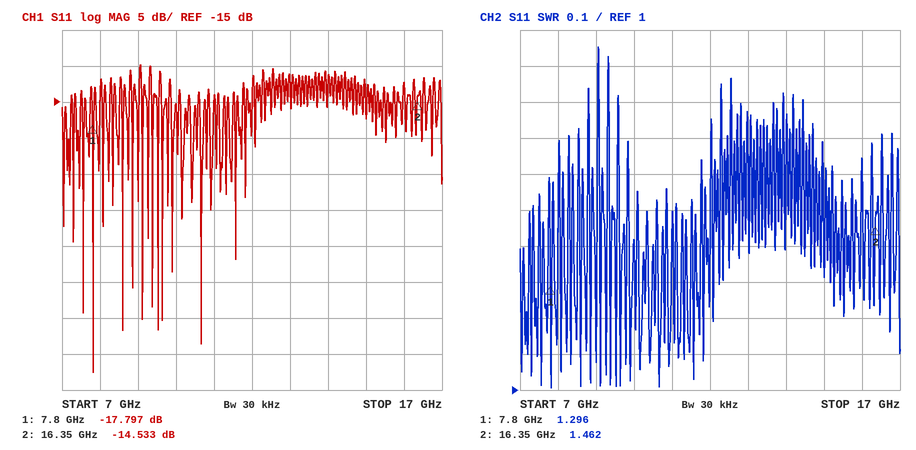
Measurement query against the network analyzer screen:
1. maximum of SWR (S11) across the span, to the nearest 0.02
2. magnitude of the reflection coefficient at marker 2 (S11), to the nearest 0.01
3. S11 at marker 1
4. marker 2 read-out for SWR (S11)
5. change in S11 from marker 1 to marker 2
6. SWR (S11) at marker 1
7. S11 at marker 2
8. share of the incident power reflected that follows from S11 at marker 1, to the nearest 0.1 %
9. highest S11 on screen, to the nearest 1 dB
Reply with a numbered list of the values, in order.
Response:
1. 1.96
2. 0.19
3. -17.797 dB
4. 1.462
5. 3.264 dB
6. 1.296
7. -14.533 dB
8. 1.7 %
9. -10 dB
